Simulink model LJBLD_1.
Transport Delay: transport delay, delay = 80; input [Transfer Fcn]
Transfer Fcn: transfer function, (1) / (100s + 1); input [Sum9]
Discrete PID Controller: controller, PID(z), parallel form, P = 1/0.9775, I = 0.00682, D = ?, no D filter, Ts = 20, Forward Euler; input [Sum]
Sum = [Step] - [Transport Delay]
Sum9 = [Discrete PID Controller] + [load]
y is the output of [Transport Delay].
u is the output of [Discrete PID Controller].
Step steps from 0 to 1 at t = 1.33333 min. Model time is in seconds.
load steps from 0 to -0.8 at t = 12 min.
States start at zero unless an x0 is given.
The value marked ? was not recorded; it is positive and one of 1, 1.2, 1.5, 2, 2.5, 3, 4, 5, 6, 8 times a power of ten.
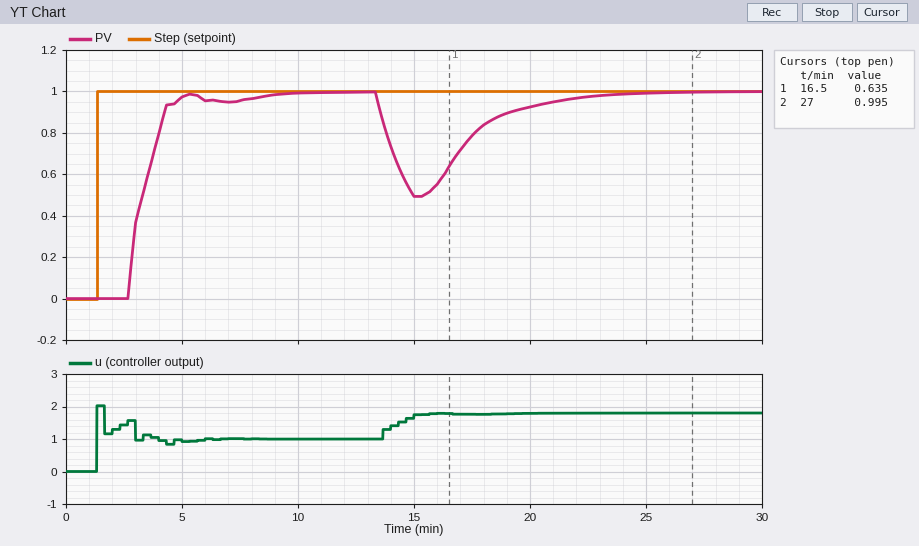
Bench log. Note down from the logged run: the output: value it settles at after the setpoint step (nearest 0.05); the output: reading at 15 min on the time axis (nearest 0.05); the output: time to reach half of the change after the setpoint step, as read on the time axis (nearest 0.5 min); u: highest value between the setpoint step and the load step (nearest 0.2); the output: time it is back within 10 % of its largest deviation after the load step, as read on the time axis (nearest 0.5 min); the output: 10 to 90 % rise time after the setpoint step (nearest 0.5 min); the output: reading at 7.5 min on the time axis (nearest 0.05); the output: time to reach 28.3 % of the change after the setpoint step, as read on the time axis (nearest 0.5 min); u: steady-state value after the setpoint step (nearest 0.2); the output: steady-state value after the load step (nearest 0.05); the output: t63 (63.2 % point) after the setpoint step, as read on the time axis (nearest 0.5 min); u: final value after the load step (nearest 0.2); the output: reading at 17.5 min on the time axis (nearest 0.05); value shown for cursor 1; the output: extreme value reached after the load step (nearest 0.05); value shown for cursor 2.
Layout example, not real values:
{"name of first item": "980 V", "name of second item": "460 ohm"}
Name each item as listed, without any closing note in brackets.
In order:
{"the output: value it settles at after the setpoint step": "1.00", "the output: reading at 15 min on the time axis": "0.50", "the output: time to reach half of the change after the setpoint step, as read on the time axis": "3.5 min", "u: highest value between the setpoint step and the load step": "2.0", "the output: time it is back within 10 % of its largest deviation after the load step, as read on the time axis": "21.0 min", "the output: 10 to 90 % rise time after the setpoint step": "1.5 min", "the output: reading at 7.5 min on the time axis": "0.95", "the output: time to reach 28.3 % of the change after the setpoint step, as read on the time axis": "3.0 min", "u: steady-state value after the setpoint step": "1.0", "the output: steady-state value after the load step": "1.00", "the output: t63 (63.2 % point) after the setpoint step, as read on the time axis": "3.5 min", "u: final value after the load step": "1.8", "the output: reading at 17.5 min on the time axis": "0.80", "value shown for cursor 1": "0.635", "the output: extreme value reached after the load step": "0.50", "value shown for cursor 2": "0.995"}
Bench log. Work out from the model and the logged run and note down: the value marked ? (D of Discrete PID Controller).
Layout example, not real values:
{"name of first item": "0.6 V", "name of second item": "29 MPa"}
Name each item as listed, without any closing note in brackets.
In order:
{"the value marked ?": "20"}
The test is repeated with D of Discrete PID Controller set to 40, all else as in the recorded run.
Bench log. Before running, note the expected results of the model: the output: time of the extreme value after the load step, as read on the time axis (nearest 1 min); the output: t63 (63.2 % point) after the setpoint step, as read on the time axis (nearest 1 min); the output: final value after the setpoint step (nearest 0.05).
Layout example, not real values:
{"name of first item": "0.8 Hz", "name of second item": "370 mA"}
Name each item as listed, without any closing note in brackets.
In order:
{"the output: time of the extreme value after the load step, as read on the time axis": "15 min", "the output: t63 (63.2 % point) after the setpoint step, as read on the time axis": "3 min", "the output: final value after the setpoint step": "1.00"}
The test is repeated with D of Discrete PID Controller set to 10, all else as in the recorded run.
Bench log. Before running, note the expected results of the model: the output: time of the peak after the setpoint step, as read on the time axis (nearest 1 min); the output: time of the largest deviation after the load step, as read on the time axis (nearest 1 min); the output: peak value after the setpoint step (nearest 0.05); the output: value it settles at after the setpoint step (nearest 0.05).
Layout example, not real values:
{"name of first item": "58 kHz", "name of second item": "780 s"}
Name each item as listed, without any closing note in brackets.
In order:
{"the output: time of the peak after the setpoint step, as read on the time axis": "6 min", "the output: time of the largest deviation after the load step, as read on the time axis": "15 min", "the output: peak value after the setpoint step": "1.05", "the output: value it settles at after the setpoint step": "1.00"}
